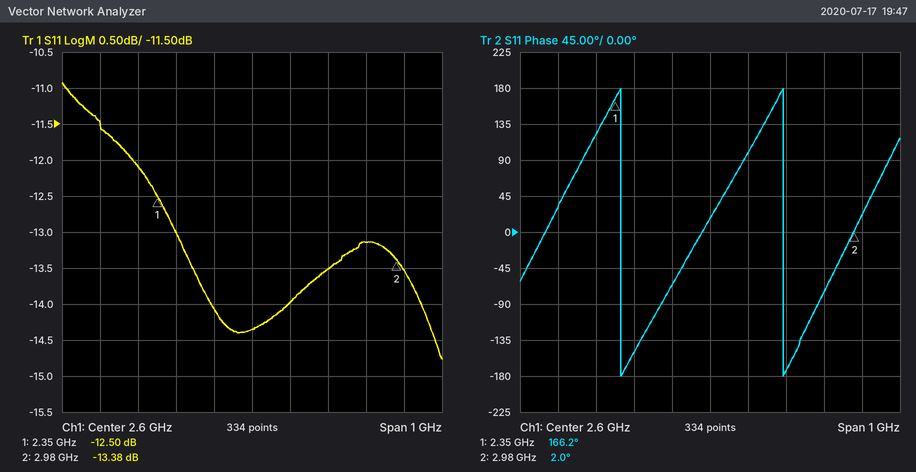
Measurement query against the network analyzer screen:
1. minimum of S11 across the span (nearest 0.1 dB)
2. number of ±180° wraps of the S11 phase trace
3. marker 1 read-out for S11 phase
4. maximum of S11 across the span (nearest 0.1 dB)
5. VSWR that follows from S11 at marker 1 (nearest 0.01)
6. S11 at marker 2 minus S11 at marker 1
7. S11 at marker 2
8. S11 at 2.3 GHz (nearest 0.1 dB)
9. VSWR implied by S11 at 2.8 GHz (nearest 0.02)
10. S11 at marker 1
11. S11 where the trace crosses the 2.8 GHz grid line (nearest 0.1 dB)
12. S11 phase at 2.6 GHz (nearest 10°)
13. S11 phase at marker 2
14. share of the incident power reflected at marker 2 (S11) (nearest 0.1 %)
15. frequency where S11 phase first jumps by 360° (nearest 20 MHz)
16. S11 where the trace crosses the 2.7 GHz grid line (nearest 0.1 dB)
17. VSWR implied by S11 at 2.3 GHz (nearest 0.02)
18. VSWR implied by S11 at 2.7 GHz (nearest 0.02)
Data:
-14.8 dB
2
166.2°
-10.9 dB
1.62
-0.88 dB
-13.38 dB
-12.1 dB
1.54
-12.50 dB
-13.5 dB
20°
2.0°
4.6 %
2.36 GHz
-14.0 dB
1.66
1.50
